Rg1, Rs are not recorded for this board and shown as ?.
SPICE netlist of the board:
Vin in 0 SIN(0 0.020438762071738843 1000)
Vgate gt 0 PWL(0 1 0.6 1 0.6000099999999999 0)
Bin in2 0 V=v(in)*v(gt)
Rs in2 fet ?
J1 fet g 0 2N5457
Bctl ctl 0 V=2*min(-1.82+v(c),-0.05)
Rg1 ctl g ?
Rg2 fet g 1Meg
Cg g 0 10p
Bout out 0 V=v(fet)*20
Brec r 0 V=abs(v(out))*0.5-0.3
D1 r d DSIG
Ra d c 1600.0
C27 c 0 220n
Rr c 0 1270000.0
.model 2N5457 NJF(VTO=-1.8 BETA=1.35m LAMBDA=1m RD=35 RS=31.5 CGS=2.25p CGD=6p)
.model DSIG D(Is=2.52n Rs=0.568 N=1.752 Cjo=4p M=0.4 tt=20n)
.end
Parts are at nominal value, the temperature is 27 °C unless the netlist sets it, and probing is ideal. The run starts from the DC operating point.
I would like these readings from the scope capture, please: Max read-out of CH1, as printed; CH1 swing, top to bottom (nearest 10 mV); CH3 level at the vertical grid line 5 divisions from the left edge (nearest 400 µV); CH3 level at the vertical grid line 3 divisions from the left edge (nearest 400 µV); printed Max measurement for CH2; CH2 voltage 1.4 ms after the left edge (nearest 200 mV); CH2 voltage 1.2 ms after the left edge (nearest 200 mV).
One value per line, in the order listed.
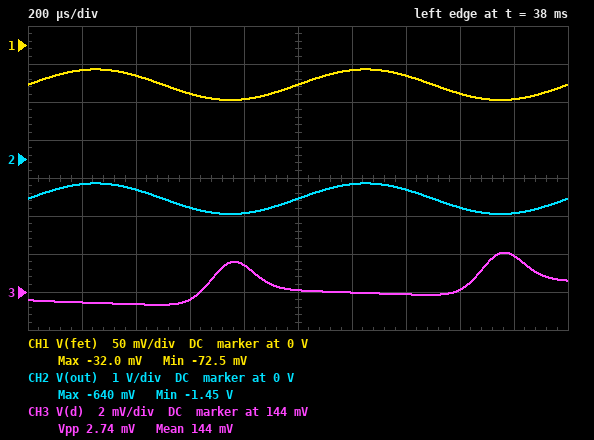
-32.0 mV
40 mV
144.0 mV
143.6 mV
-640 mV
-800 mV
-600 mV
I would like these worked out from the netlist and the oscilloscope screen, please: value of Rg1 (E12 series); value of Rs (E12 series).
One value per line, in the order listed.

390 kΩ
22 kΩ
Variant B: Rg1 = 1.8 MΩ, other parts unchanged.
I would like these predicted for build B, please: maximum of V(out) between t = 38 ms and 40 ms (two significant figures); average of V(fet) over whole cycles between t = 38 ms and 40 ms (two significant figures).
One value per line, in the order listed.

-5.8 mV
-1.0 mV
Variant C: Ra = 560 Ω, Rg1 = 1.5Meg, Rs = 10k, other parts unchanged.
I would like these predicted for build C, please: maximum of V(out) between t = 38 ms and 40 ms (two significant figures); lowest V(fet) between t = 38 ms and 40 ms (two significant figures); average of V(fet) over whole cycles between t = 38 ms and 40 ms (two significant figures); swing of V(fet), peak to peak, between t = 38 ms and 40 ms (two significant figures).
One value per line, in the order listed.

12 mV
-3.6 mV
-1.5 mV
4.2 mV
